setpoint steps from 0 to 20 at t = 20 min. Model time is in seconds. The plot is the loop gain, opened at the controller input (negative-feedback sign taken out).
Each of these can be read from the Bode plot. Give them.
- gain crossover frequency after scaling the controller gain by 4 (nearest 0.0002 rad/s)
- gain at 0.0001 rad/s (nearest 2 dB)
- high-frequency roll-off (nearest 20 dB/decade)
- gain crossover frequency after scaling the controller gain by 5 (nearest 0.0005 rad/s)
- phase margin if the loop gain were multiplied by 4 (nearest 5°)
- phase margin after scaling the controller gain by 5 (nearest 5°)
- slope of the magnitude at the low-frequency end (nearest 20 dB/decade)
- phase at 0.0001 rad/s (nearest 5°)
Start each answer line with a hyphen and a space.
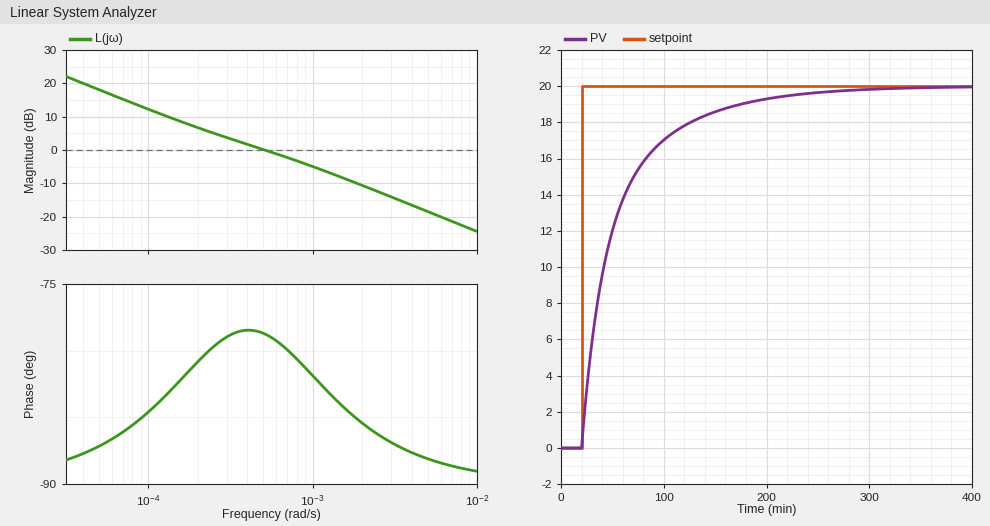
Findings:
- 0.0024 rad/s
- 12 dB
- -20 dB/decade
- 0.0030 rad/s
- 95°
- 95°
- -20 dB/decade
- -85°
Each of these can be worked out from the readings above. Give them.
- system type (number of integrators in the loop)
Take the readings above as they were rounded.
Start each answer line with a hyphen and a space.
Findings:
- 1
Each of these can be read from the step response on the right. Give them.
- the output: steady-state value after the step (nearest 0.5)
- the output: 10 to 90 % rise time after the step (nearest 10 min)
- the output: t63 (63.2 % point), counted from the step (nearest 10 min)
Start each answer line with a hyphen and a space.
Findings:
- 20.0
- 100 min
- 30 min
